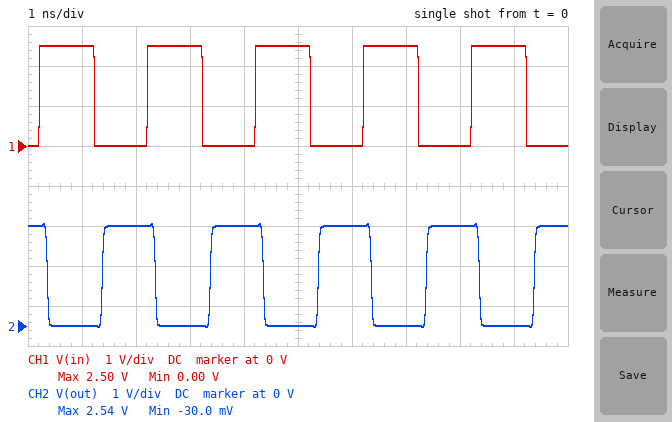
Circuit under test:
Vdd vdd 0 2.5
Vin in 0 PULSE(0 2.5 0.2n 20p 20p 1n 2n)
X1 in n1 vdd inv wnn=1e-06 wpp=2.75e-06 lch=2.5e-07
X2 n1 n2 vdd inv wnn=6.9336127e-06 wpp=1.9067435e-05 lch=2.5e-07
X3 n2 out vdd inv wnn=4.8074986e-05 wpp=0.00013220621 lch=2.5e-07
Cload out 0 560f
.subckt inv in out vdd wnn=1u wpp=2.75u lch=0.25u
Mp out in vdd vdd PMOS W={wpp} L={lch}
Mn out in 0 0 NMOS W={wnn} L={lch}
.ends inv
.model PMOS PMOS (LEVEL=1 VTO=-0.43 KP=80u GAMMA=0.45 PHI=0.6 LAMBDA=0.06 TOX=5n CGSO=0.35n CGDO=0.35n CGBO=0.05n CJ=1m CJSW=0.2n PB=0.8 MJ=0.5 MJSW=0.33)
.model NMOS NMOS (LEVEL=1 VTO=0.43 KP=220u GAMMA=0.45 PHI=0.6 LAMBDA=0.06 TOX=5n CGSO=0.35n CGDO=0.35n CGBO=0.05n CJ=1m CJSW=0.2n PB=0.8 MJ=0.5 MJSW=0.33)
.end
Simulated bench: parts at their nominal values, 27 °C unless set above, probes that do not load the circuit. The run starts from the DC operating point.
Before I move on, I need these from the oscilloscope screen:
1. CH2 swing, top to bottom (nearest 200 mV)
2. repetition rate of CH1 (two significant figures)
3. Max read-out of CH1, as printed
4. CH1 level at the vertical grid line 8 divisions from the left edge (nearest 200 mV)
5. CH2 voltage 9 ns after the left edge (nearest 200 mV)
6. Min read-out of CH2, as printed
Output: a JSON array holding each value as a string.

["2.6 V", "500 MHz", "2.50 V", "0 V", "0 V", "-30.0 mV"]
